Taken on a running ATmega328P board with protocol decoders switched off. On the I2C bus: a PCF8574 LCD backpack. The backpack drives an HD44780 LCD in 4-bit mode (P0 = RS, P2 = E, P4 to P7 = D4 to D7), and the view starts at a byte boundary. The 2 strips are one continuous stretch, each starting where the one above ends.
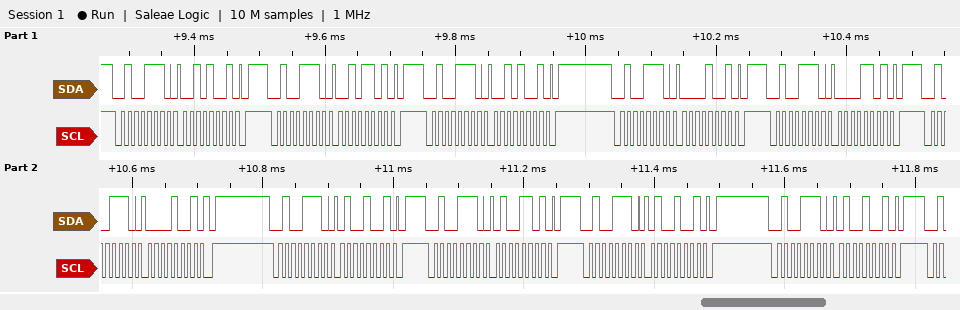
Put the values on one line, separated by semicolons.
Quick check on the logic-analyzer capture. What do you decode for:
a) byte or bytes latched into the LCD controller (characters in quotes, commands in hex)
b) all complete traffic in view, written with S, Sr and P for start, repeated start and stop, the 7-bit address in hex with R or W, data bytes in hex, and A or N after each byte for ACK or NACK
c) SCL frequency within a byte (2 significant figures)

' '; S 27W A 29 A P S 27W A 2D A P S 27W A 29 A P S 27W A 09 A P S 27W A 0D A P S 27W A 09 A P S 27W A 49 A P S 27W A 4D A P S 27W A 49 A P S 27W A 49 A P; 100 kHz
